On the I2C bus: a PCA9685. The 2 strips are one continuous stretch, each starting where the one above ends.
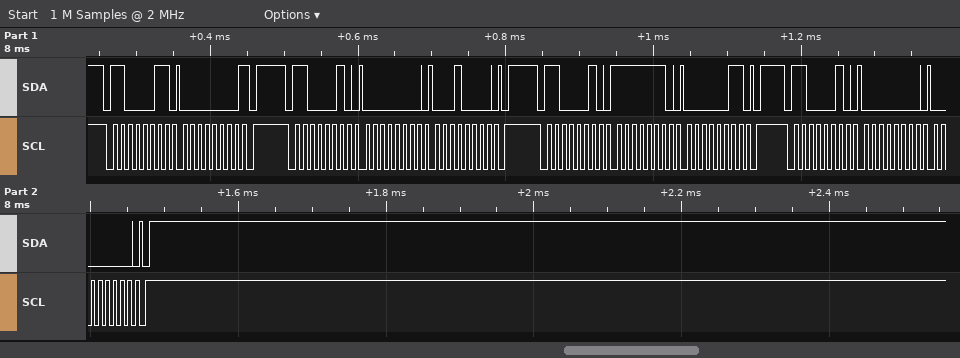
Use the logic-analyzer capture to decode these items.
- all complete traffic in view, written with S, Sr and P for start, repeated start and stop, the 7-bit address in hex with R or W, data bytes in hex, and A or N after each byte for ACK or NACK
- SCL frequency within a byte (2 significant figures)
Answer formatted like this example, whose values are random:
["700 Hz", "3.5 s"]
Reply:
["S 61R A 00 N P S 61W A 00 A 10 A P S 61W A FE A 03 A P S 61W A 00 A 00 A P", "100 kHz"]
